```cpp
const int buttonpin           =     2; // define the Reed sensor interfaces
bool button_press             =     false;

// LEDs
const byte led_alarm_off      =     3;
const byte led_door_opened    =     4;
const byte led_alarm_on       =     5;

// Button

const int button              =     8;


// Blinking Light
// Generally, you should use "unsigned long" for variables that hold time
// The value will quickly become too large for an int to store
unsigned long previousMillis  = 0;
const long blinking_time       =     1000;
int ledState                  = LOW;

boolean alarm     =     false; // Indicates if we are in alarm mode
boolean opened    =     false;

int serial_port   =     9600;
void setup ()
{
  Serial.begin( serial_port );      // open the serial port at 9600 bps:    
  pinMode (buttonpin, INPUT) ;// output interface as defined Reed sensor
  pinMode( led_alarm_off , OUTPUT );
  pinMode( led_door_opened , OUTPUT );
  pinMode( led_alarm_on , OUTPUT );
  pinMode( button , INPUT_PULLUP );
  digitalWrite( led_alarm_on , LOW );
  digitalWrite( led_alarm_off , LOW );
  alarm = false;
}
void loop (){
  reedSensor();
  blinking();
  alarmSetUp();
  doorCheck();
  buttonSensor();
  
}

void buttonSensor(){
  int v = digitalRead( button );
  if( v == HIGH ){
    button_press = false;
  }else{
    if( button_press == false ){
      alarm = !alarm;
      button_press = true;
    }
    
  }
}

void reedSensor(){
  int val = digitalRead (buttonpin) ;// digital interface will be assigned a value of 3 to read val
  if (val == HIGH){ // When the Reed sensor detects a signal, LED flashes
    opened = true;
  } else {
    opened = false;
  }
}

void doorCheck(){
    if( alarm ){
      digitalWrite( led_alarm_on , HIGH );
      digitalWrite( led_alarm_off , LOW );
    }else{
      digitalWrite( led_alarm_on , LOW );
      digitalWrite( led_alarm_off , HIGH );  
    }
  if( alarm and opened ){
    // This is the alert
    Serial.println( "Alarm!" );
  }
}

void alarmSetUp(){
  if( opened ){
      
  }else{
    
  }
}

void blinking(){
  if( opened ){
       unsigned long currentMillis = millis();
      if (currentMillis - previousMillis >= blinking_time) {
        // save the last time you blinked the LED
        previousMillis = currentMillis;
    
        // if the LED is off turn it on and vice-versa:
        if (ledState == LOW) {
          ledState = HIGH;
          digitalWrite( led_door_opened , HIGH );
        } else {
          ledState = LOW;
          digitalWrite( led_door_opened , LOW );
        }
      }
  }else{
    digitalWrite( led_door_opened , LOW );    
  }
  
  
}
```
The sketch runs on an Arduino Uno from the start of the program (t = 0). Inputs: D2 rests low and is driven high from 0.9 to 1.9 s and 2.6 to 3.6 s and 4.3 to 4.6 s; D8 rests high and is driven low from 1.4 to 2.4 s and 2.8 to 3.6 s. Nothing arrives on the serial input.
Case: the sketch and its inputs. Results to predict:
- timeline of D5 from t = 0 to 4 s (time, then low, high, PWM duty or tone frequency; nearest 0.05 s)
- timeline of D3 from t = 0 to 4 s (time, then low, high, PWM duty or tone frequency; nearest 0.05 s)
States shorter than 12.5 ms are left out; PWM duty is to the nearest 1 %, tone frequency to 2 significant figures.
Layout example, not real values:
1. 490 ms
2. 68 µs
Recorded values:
1. 0 s low; 1.4 s high; 2.8 s low
2. 0 s high; 1.4 s low; 2.8 s high
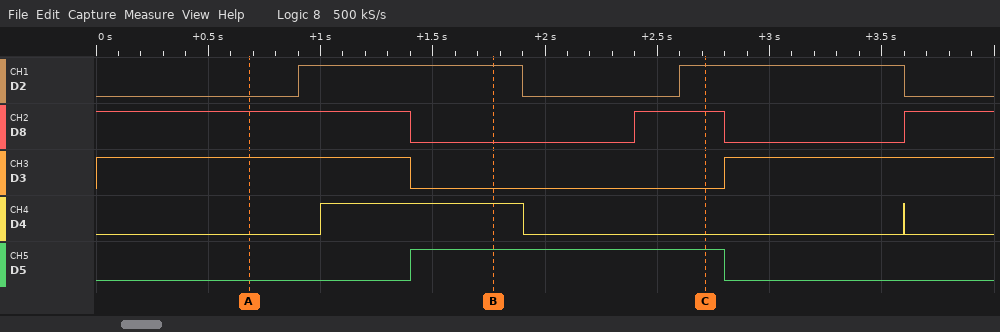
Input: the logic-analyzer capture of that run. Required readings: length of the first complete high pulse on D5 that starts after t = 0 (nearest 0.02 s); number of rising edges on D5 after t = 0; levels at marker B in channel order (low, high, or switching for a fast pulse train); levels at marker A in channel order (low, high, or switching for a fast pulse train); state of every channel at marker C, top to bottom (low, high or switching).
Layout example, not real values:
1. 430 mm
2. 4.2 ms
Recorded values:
1. 1.40 s
2. 1
3. D2 high, D8 low, D3 low, D4 high, D5 high
4. D2 low, D8 high, D3 high, D4 low, D5 low
5. D2 high, D8 high, D3 low, D4 low, D5 high
